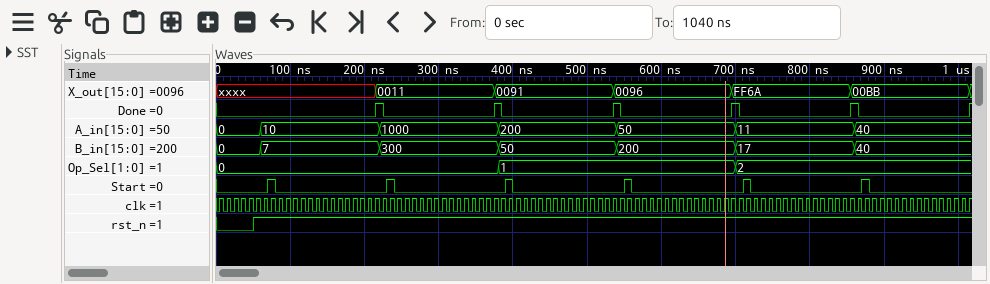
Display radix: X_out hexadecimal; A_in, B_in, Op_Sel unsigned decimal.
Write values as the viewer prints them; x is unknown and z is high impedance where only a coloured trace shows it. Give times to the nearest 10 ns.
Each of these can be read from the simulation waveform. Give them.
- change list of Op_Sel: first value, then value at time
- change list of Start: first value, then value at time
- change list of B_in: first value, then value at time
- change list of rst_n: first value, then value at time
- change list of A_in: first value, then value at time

0, 1 at 380 ns, 2 at 700 ns
0, 1 at 70 ns, 0 at 80 ns, 1 at 230 ns, 0 at 240 ns, 1 at 390 ns, 0 at 400 ns, 1 at 550 ns, 0 at 560 ns, 1 at 710 ns, 0 at 720 ns, 1 at 870 ns, 0 at 880 ns
0, 7 at 60 ns, 300 at 220 ns, 50 at 380 ns, 200 at 540 ns, 17 at 700 ns, 40 at 860 ns
0, 1 at 50 ns
0, 10 at 60 ns, 1000 at 220 ns, 200 at 380 ns, 50 at 540 ns, 11 at 700 ns, 40 at 860 ns
